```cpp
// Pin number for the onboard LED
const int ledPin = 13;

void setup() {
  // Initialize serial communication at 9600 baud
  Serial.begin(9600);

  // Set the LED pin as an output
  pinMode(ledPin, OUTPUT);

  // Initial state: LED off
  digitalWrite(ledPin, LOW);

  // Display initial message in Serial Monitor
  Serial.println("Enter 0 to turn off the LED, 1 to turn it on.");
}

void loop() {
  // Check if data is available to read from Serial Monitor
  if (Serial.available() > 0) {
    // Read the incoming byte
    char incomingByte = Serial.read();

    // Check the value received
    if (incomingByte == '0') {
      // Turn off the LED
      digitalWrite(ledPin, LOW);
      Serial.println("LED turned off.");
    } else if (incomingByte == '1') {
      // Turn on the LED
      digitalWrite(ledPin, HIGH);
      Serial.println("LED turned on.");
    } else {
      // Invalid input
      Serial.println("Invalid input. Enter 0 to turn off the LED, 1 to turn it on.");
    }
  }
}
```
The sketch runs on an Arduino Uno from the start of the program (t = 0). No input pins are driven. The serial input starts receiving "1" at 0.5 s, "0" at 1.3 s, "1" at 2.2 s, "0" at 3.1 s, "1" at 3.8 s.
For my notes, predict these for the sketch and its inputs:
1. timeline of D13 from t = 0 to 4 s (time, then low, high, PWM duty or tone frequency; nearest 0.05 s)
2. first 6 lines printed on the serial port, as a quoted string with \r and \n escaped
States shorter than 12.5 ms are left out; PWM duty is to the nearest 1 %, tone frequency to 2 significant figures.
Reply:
0 s low; 0.5 s high; 1.3 s low; 2.2 s high; 3.1 s low; 3.8 s high
"Enter 0 to turn off the LED, 1 to turn it on.\r\nLED turned on.\r\nLED turned off.\r\nLED turned on.\r\nLED turned off.\r\nLED turned on.\r\n"
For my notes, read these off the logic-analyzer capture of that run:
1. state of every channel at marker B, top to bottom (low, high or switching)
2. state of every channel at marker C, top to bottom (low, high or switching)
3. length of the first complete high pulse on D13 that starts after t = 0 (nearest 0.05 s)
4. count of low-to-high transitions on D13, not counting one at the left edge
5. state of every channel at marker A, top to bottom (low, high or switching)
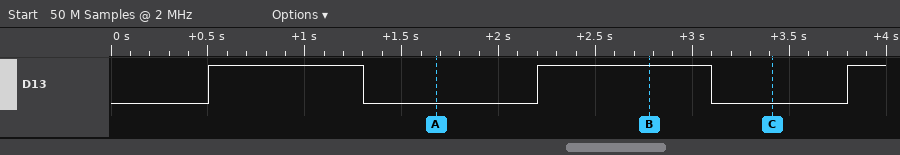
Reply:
D13 high
D13 low
0.80 s
3
D13 low
